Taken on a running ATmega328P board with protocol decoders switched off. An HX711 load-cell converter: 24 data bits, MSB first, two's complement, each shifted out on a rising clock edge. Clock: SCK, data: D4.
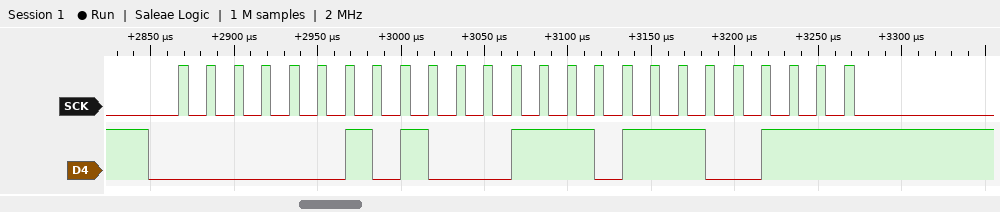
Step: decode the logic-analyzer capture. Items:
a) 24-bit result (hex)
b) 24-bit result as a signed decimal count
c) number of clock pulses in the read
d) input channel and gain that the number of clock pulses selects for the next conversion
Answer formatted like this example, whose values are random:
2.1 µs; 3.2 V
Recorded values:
0x028EE7; 167655; 25; channel A, gain 128
